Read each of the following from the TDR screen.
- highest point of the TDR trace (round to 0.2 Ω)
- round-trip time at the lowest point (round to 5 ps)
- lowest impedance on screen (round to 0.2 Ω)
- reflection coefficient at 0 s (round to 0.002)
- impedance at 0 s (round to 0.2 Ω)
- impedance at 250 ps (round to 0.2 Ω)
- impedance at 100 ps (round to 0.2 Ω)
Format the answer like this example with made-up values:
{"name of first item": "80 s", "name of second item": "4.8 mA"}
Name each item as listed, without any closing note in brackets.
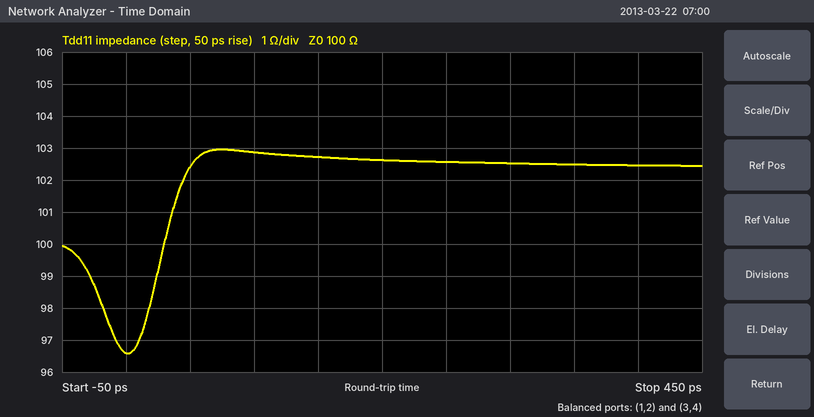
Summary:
{"highest point of the TDR trace": "103.0 Ω", "round-trip time at the lowest point": "0 ps", "lowest impedance on screen": "96.6 Ω", "reflection coefficient at 0 s": "-0.018", "impedance at 0 s": "96.6 Ω", "impedance at 250 ps": "102.6 Ω", "impedance at 100 ps": "102.8 Ω"}
